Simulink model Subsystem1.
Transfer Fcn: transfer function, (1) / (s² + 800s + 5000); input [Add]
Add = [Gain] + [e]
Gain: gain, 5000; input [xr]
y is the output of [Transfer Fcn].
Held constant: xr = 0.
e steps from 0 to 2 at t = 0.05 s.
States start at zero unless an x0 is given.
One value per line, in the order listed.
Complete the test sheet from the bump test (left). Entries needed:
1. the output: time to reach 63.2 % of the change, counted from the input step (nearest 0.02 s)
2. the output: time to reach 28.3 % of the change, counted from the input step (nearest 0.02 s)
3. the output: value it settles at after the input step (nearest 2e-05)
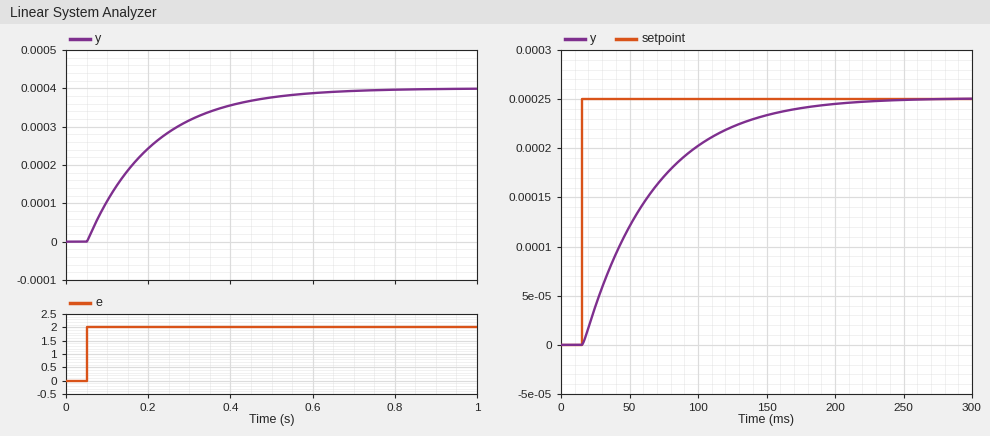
0.16 s
0.06 s
0.00040
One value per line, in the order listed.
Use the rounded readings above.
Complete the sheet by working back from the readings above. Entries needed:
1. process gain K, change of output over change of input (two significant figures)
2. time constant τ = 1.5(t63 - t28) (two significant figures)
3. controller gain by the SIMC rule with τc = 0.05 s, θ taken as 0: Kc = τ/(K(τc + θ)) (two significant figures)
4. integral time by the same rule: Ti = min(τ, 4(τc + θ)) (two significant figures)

0.00020
0.15 s
15000
0.15 s
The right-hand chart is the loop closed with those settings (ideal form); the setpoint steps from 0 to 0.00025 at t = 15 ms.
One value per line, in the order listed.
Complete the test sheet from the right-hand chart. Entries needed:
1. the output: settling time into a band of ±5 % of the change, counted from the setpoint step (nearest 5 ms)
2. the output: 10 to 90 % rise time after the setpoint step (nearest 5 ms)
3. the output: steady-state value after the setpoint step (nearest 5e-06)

145 ms
110 ms
0.000250
